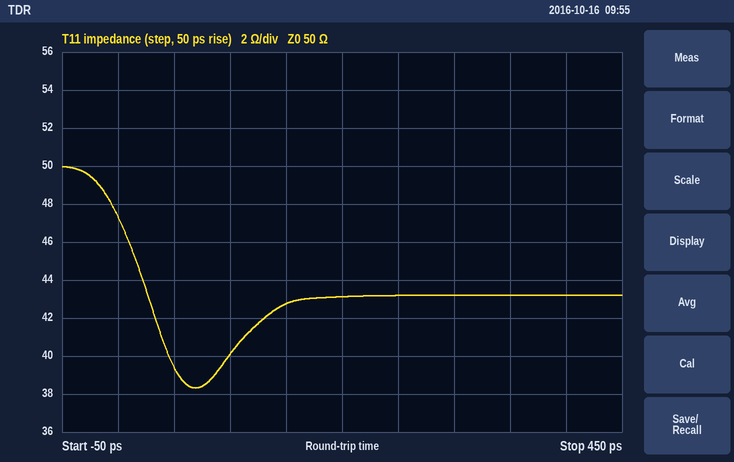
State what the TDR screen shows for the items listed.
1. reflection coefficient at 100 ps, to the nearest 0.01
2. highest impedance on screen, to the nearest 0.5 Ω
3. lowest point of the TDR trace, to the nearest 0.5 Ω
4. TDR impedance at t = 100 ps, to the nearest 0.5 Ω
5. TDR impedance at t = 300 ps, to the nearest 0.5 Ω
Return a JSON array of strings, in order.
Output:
["-0.11", "50.0 Ω", "38.5 Ω", "40.0 Ω", "43.0 Ω"]
